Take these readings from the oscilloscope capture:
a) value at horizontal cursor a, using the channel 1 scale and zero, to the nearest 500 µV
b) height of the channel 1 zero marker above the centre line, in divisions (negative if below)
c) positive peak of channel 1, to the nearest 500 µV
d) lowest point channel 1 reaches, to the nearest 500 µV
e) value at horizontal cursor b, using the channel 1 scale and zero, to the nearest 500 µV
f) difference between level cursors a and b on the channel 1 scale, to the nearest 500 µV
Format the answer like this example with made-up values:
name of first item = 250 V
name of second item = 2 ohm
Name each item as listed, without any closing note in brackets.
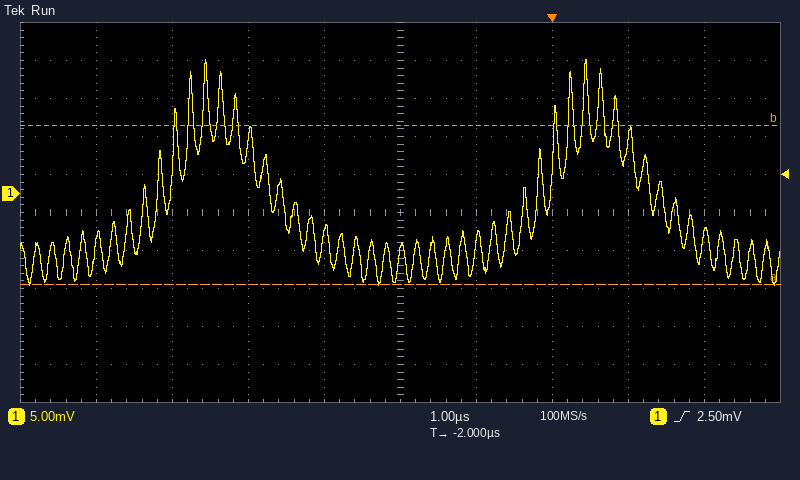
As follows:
value at horizontal cursor a, using the channel 1 scale and zero, to the nearest 500 µV = -12.0 mV
height of the channel 1 zero marker above the centre line, in divisions = +0.5 div
positive peak of channel 1, to the nearest 500 µV = 17.5 mV
lowest point channel 1 reaches, to the nearest 500 µV = -12.0 mV
value at horizontal cursor b, using the channel 1 scale and zero, to the nearest 500 µV = 9.0 mV
difference between level cursors a and b on the channel 1 scale, to the nearest 500 µV = 21.0 mV
